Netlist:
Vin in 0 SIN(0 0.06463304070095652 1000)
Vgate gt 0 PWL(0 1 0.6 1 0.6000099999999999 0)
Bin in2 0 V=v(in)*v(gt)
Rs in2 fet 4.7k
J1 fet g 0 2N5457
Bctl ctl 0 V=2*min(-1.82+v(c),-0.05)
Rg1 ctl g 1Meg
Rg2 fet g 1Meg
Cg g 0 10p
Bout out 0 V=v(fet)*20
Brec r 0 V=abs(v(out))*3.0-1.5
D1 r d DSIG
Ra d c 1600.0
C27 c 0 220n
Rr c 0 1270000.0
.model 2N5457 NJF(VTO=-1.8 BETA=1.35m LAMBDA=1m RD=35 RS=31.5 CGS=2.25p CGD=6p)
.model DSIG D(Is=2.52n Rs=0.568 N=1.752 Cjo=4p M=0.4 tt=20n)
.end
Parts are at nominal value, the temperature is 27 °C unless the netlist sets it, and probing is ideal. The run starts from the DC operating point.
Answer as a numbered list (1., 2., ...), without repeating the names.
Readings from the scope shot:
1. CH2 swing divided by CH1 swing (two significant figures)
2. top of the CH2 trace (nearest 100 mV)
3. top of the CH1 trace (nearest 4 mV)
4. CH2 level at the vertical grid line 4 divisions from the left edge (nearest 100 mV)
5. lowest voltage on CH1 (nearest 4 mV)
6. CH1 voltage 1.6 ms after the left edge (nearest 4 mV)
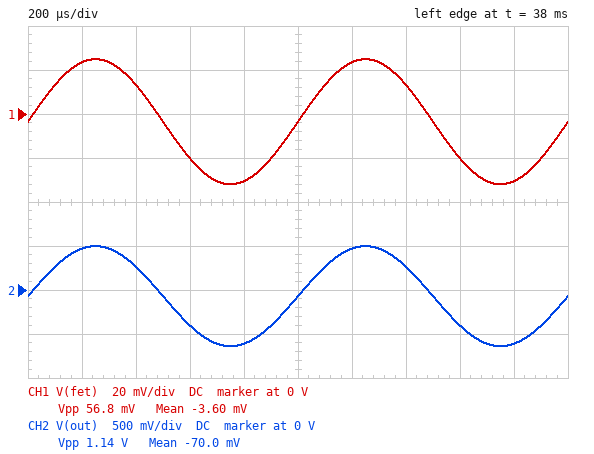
1. 20
2. 500 mV
3. 24 mV
4. -600 mV
5. -32 mV
6. -20 mV
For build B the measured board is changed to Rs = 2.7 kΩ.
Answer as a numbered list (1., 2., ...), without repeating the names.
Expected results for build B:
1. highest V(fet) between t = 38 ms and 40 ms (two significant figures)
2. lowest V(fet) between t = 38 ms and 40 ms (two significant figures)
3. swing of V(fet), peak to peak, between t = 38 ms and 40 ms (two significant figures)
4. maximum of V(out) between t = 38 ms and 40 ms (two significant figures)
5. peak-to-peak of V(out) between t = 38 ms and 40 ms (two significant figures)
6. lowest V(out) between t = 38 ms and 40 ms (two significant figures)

1. 29 mV
2. -33 mV
3. 62 mV
4. 580 mV
5. 1.2 V
6. -660 mV
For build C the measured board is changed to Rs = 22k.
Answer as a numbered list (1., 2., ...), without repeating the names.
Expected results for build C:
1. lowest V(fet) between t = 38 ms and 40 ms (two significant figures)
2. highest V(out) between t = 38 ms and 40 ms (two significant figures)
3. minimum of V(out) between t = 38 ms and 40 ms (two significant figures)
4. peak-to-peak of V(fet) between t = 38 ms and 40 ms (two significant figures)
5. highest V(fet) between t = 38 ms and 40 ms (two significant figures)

1. -30 mV
2. 150 mV
3. -600 mV
4. 38 mV
5. 7.6 mV
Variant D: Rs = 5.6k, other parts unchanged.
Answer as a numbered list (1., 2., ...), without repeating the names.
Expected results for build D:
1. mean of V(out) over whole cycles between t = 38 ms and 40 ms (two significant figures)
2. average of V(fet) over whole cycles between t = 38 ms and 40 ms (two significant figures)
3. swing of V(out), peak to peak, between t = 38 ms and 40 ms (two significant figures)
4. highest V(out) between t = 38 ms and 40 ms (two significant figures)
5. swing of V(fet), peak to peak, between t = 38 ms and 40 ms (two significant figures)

1. -82 mV
2. -4.1 mV
3. 1.1 V
4. 470 mV
5. 55 mV
